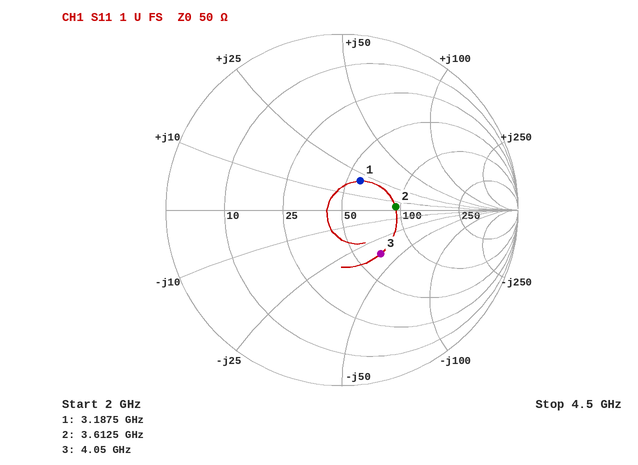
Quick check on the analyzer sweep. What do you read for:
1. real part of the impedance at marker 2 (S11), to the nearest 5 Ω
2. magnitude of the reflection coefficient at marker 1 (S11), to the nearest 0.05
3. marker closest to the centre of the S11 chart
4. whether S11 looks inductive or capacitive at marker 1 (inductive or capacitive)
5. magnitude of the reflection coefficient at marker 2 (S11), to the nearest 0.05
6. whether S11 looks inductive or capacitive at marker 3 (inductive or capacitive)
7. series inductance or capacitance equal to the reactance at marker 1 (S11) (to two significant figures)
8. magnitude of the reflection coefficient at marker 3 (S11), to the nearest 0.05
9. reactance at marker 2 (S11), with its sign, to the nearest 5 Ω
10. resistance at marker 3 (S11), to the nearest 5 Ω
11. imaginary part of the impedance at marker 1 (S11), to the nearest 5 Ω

95 Ω
0.20
marker 1
inductive
0.30
capacitive
1.0 nH
0.35
+5 Ω
65 Ω
+20 Ω
